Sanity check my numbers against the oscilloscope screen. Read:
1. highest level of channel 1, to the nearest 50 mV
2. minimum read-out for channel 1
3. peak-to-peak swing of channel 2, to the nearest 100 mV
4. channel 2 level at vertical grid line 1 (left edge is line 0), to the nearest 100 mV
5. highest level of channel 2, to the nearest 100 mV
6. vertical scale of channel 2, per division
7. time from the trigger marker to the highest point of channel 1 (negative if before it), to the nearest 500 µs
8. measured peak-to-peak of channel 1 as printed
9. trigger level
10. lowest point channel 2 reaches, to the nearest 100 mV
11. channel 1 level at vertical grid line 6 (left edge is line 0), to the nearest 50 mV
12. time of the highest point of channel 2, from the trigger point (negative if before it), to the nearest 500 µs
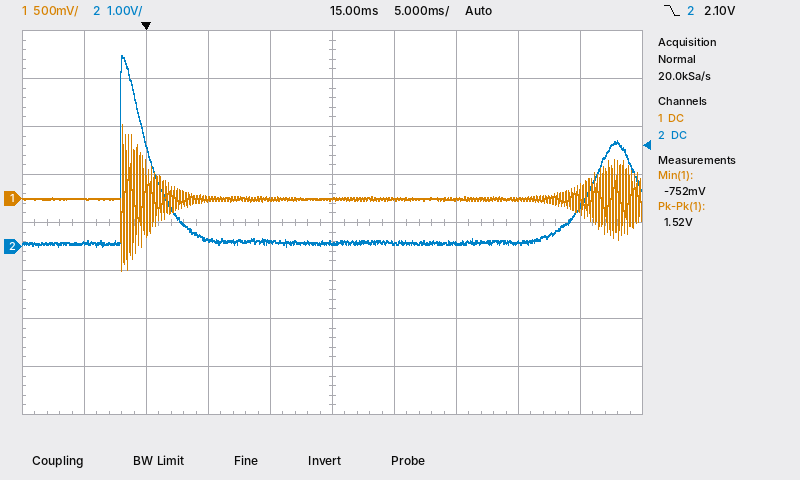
750 mV
-752 mV
4.0 V
100 mV
4.0 V
1 V
-2.0 ms
1.52 V
2.10 V
0.0 V
0 mV
-2.0 ms
